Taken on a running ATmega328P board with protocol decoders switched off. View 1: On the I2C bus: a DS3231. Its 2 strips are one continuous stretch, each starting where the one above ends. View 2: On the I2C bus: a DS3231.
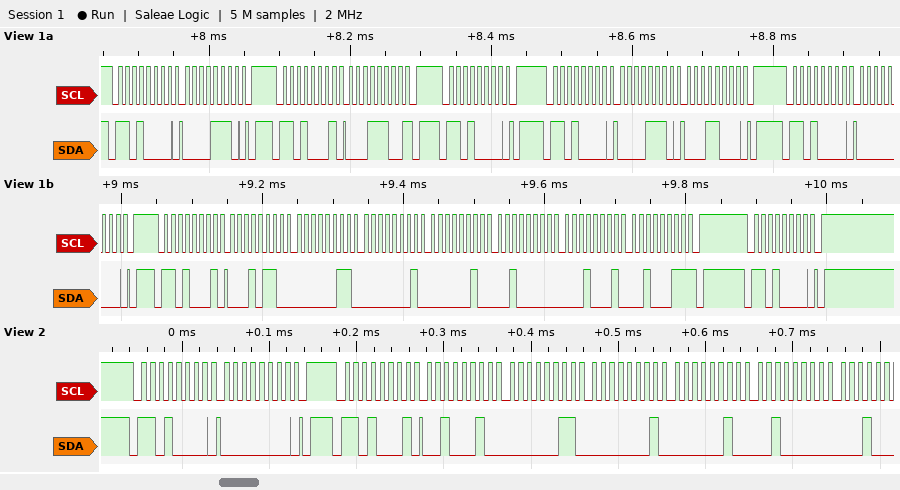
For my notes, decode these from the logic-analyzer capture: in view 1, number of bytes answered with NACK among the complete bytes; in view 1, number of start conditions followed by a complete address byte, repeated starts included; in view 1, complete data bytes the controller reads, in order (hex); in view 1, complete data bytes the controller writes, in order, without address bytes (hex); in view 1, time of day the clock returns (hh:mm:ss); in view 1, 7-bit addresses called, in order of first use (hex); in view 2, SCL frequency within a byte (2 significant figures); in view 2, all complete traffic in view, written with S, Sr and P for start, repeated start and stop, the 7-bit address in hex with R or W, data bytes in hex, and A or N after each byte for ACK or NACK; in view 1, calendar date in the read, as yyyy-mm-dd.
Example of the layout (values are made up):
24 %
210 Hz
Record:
2
7
1C 16 03 01 02 20 11 23
0E 0E 18 00
01:03:16
0x68
100 kHz
S 68W A 00 A P S 68R A 22 A 03 A 01 A 02 A 20 A
2023-11-20
